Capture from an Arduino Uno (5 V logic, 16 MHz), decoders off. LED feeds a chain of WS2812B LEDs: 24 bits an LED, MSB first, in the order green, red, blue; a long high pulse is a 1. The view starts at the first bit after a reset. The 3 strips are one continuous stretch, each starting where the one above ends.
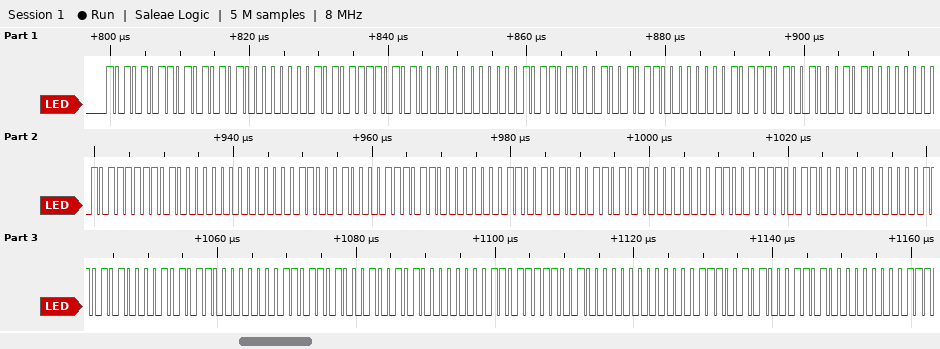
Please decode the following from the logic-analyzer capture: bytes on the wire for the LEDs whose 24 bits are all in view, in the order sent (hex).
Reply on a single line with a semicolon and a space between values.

AB 55 00 AF 50 00 B4 4B 00 BA 45 00 BF 40 00 C4 3B 00 CA 35 00 CF 30 00 D4 2B 00 DA 25 00 DF 20 00 E5 1A 00
